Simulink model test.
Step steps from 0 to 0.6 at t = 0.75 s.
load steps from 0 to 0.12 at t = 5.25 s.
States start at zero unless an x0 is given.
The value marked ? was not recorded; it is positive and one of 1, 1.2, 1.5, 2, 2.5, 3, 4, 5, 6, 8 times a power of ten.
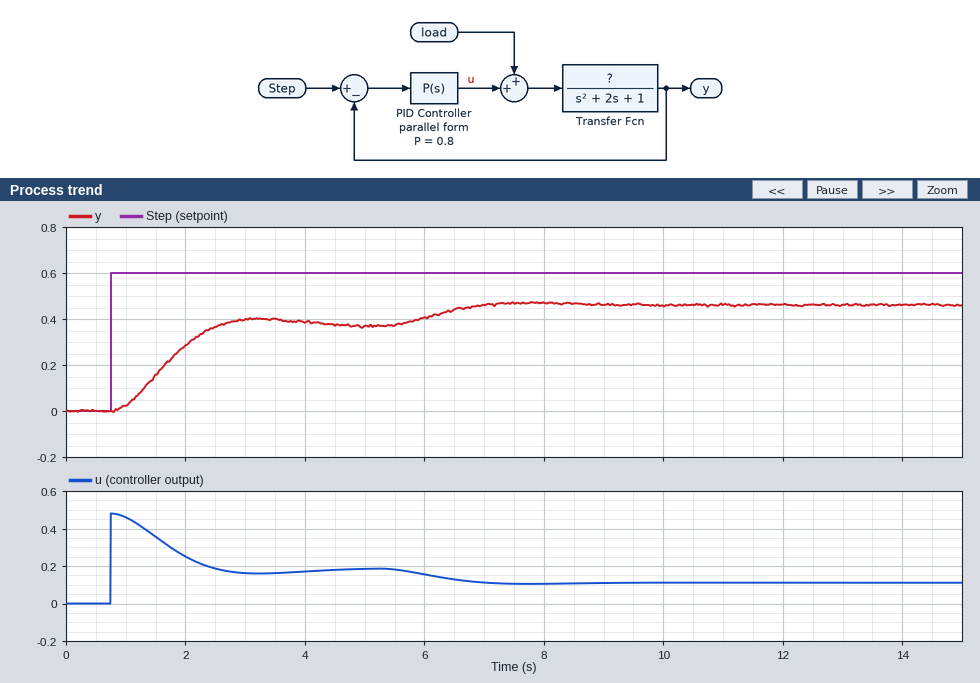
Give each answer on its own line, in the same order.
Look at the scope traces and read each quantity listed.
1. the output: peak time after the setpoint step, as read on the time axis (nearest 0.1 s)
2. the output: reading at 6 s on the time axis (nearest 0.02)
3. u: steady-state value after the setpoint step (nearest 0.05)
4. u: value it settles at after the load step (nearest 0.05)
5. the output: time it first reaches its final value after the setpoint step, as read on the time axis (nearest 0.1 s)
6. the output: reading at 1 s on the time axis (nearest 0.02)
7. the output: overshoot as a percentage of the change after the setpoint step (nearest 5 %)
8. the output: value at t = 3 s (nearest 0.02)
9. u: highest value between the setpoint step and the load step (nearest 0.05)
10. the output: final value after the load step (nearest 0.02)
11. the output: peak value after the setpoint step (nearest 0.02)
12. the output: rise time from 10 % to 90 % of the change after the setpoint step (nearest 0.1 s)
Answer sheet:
3.2 s
0.40
0.20
0.10
2.5 s
0.02
10 %
0.40
0.50
0.46
0.40
1.2 s
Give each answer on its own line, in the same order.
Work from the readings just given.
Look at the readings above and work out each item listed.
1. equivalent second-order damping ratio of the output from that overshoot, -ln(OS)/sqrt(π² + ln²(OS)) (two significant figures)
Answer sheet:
0.59
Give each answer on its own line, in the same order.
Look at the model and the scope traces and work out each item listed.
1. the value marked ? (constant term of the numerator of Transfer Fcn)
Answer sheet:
2
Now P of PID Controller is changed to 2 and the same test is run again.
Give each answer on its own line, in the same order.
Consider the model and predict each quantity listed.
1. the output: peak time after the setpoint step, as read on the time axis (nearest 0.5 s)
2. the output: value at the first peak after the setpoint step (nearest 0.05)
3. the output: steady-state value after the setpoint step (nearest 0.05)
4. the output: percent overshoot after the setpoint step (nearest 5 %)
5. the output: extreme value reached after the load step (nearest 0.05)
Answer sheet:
2.5 s
0.60
0.50
20 %
0.55
